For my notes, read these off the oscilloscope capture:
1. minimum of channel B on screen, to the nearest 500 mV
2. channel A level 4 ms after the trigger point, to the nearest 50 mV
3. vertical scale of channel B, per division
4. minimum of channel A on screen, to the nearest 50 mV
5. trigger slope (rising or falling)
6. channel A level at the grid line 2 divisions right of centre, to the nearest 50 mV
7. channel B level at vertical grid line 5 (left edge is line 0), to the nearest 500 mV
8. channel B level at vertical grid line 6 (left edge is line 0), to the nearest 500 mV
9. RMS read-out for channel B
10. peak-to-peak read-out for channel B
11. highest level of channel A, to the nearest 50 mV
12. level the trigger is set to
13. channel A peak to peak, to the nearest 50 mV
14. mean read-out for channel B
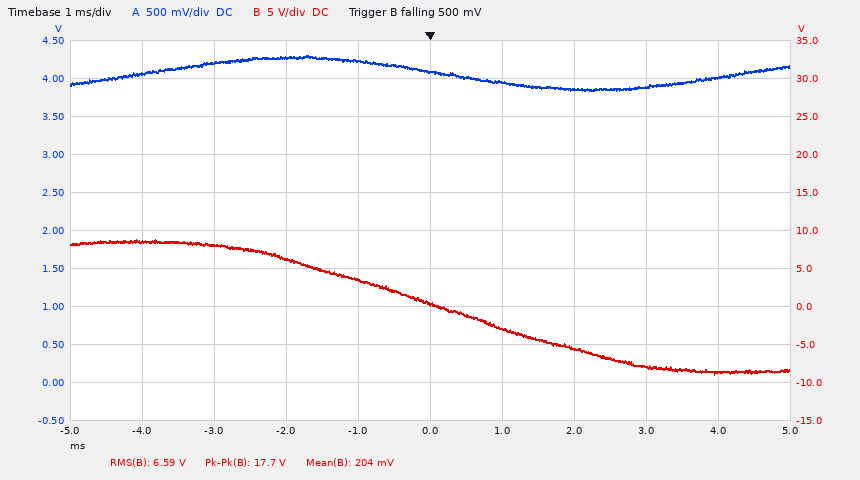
-9.0 V
4.00 V
5 V
3.85 V
falling
3.85 V
500 mV
-3.0 V
6.59 V
17.7 V
4.30 V
500 mV
450 mV
204 mV
